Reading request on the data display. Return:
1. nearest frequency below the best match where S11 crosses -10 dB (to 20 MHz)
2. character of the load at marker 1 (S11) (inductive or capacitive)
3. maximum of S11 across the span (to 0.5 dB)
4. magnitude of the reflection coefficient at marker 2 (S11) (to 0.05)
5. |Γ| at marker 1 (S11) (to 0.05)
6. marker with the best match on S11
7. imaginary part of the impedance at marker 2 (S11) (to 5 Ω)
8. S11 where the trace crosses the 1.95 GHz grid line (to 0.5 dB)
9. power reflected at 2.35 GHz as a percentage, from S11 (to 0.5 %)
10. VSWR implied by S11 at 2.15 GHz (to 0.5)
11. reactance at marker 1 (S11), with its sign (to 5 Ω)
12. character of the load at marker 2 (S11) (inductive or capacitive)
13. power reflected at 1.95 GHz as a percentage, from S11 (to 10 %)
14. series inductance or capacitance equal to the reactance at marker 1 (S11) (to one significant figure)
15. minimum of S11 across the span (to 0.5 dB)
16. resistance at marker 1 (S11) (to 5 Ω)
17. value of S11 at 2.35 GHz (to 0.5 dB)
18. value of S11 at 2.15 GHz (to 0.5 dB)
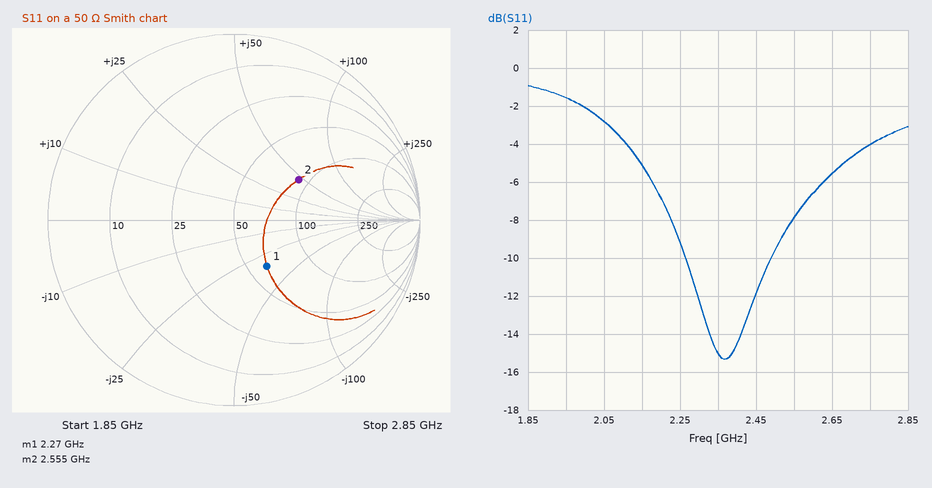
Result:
2.26 GHz
capacitive
-1.0 dB
0.40
0.30
marker 1
+45 Ω
-1.5 dB
3.0 %
3.5
-35 Ω
inductive
70 %
2 pF
-15.5 dB
60 Ω
-15.0 dB
-5.0 dB
